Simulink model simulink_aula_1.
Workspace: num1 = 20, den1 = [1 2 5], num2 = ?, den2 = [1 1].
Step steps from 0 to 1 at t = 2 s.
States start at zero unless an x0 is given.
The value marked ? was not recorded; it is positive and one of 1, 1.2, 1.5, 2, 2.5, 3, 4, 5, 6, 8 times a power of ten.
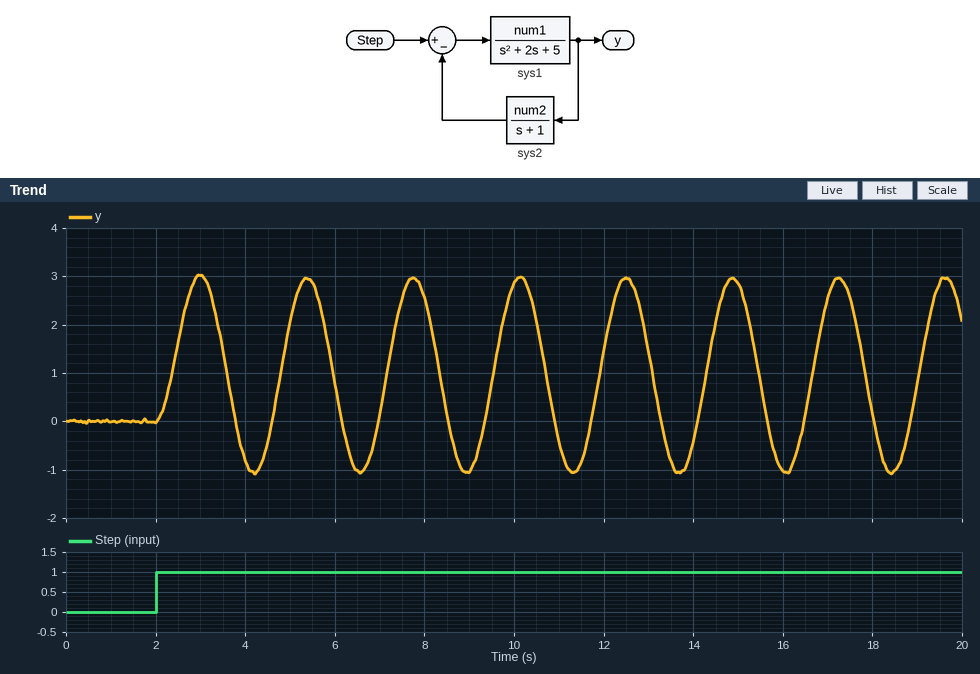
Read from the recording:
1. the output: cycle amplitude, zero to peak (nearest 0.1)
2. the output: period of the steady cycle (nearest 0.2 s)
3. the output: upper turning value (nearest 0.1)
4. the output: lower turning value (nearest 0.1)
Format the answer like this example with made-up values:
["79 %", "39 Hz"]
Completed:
["2.0", "2.4 s", "3.0", "-1.1"]
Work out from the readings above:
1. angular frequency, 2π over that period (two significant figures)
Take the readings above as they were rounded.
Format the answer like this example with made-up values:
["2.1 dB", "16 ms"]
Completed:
["2.6 rad/s"]
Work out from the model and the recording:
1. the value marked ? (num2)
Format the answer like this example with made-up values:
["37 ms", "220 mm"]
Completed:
["0.8"]
